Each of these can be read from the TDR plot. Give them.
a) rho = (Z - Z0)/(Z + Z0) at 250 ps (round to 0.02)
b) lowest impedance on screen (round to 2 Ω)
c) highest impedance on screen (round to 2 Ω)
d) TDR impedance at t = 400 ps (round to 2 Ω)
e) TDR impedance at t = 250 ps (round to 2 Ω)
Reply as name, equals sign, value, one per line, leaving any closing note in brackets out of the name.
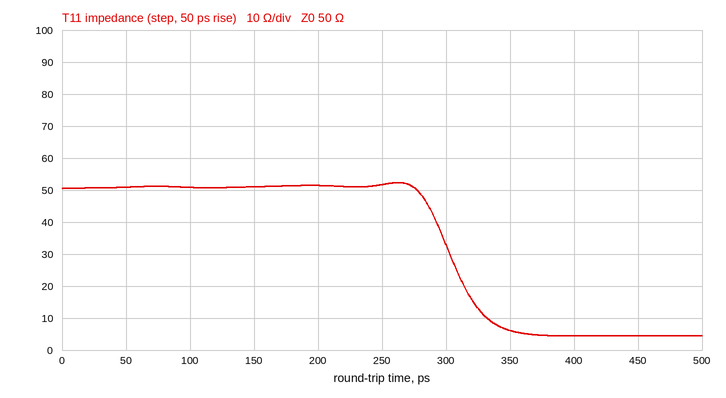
rho = (Z - Z0)/(Z + Z0) at 250 ps = +0.02
lowest impedance on screen = 4 Ω
highest impedance on screen = 52 Ω
TDR impedance at t = 400 ps = 4 Ω
TDR impedance at t = 250 ps = 52 Ω
